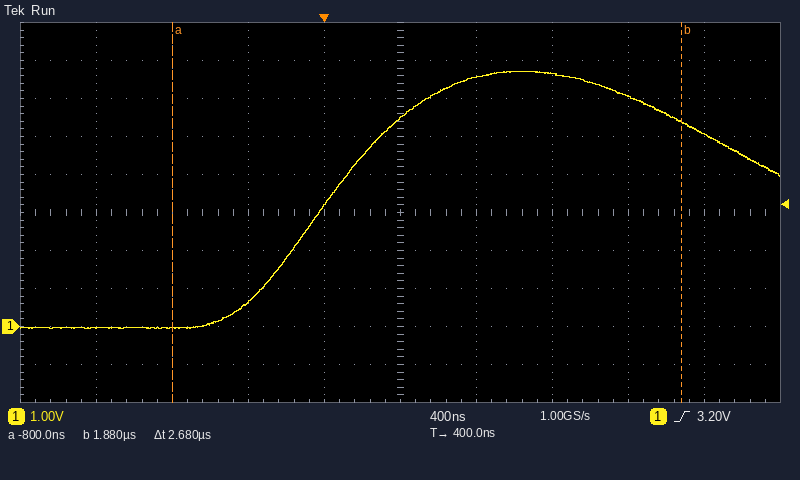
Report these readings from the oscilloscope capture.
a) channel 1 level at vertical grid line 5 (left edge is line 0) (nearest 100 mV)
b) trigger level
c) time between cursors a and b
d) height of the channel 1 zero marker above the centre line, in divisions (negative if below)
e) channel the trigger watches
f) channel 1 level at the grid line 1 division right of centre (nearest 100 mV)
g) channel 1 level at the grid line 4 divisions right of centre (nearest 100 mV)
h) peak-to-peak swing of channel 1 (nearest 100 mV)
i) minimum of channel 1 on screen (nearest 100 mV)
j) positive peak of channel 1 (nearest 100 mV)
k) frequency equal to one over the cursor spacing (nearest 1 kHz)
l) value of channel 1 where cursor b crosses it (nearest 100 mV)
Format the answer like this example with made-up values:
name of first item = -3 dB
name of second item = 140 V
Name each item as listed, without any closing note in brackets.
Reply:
channel 1 level at vertical grid line 5 (left edge is line 0) = 5.5 V
trigger level = 3.20 V
time between cursors a and b = 2.68 µs
height of the channel 1 zero marker above the centre line, in divisions = -3.0 div
channel the trigger watches = channel 1
channel 1 level at the grid line 1 division right of centre = 6.6 V
channel 1 level at the grid line 4 divisions right of centre = 5.1 V
peak-to-peak swing of channel 1 = 6.8 V
minimum of channel 1 on screen = -100 mV
positive peak of channel 1 = 6.7 V
frequency equal to one over the cursor spacing = 373 kHz
value of channel 1 where cursor b crosses it = 5.4 V
